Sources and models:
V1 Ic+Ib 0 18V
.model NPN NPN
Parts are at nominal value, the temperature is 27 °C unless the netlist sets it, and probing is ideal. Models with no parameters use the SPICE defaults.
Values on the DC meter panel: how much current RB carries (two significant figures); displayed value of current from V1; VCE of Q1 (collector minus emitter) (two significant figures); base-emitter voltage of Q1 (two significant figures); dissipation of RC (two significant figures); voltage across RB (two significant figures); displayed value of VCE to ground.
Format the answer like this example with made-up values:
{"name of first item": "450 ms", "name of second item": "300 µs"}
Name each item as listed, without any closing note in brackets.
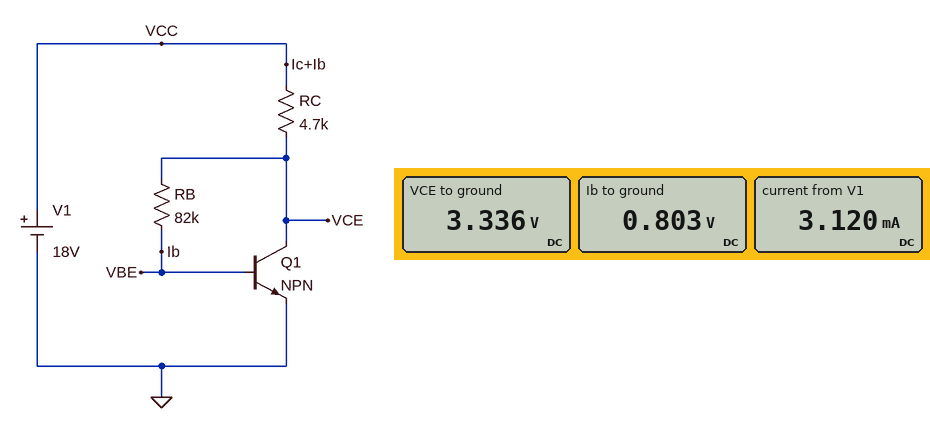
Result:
{"how much current RB carries": "31 µA", "displayed value of current from V1": "3.120 mA", "VCE of Q1 (collector minus emitter)": "3.3 V", "base-emitter voltage of Q1": "800 mV", "dissipation of RC": "46 mW", "voltage across RB": "2.5 V", "displayed value of VCE to ground": "3.336 V"}
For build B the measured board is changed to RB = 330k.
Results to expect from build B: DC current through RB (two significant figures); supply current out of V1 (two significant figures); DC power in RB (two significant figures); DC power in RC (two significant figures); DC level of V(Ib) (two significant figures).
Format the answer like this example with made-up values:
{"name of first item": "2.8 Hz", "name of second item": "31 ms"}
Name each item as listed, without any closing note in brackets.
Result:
{"DC current through RB": "21 µA", "supply current out of V1": "2.2 mA", "DC power in RB": "150 µW", "DC power in RC": "22 mW", "DC level of V(Ib)": "790 mV"}
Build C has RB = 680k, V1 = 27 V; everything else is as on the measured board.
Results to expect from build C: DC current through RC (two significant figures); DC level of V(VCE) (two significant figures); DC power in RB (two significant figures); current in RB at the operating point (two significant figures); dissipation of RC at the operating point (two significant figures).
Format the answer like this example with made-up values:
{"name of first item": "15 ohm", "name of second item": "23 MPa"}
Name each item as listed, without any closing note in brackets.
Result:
{"DC current through RC": "2.3 mA", "DC level of V(VCE)": "16 V", "DC power in RB": "350 µW", "current in RB at the operating point": "23 µA", "dissipation of RC at the operating point": "25 mW"}
